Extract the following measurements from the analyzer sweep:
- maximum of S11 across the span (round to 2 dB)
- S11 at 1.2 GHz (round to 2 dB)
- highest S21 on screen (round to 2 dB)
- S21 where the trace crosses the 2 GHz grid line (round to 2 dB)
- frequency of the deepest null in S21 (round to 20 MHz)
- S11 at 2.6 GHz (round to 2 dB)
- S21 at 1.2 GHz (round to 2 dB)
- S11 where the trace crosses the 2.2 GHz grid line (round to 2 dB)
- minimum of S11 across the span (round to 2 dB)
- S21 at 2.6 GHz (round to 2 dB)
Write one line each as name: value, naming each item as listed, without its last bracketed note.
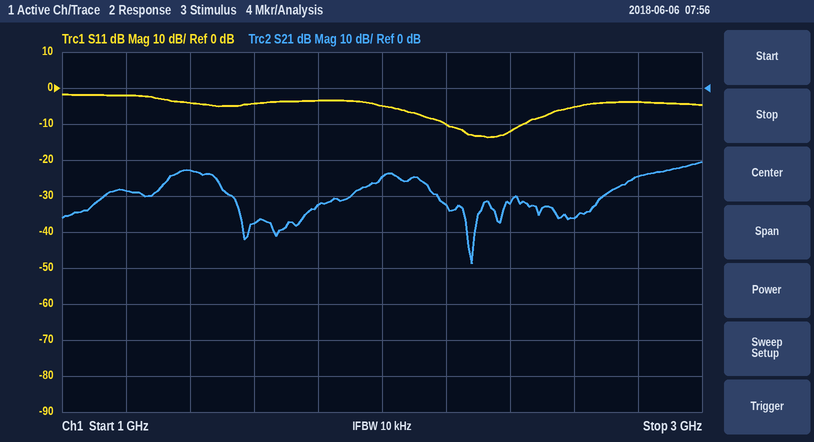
maximum of S11 across the span: -2 dB
S11 at 1.2 GHz: -2 dB
highest S21 on screen: -20 dB
S21 where the trace crosses the 2 GHz grid line: -24 dB
frequency of the deepest null in S21: 2.28 GHz
S11 at 2.6 GHz: -6 dB
S21 at 1.2 GHz: -28 dB
S11 where the trace crosses the 2.2 GHz grid line: -10 dB
minimum of S11 across the span: -14 dB
S21 at 2.6 GHz: -36 dB
